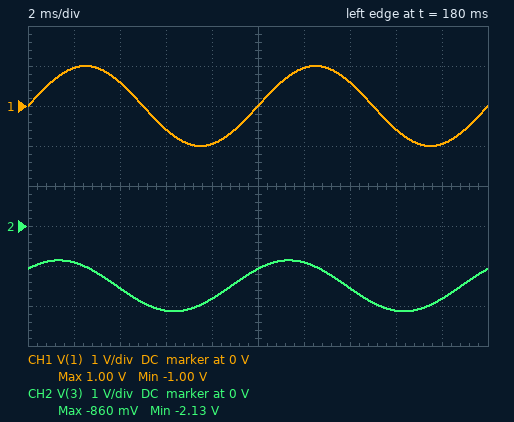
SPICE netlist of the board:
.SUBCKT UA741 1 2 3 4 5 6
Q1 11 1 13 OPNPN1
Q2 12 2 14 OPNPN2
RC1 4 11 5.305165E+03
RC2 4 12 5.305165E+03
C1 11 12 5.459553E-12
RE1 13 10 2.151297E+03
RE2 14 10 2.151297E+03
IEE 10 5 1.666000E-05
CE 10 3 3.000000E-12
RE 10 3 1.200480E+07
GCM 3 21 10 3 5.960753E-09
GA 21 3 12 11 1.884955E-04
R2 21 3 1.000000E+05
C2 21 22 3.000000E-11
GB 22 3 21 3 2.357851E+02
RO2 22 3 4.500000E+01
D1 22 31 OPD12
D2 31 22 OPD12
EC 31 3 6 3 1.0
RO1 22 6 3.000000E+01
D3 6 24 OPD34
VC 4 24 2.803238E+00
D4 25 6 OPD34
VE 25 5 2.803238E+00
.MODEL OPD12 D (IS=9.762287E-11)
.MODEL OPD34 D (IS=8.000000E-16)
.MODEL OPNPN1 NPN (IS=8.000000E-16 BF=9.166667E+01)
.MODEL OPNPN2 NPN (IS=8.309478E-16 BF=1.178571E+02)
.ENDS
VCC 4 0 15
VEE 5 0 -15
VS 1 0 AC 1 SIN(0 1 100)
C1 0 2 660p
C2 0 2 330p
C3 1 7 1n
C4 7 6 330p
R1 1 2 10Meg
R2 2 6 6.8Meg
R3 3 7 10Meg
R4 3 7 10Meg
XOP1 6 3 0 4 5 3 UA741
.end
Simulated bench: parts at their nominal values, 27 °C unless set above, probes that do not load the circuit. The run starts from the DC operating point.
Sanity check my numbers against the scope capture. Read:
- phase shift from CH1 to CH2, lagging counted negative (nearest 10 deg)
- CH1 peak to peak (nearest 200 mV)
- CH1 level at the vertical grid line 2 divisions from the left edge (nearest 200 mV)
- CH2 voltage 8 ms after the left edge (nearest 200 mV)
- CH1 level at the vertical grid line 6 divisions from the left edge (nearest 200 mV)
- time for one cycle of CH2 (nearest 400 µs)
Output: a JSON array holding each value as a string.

["40 deg", "2.0 V", "600 mV", "-1.8 V", "1.0 V", "10.0 ms"]
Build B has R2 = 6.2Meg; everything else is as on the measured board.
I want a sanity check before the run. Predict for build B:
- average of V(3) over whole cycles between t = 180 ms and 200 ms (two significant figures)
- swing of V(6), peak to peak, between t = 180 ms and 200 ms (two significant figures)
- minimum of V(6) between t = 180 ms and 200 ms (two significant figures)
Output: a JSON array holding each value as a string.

["-1.4 V", "1.2 V", "-2.0 V"]
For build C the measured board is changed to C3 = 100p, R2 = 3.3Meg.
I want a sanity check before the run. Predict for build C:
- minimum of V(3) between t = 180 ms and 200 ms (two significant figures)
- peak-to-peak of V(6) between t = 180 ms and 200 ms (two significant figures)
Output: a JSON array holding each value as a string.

["-1.2 V", "26 mV"]
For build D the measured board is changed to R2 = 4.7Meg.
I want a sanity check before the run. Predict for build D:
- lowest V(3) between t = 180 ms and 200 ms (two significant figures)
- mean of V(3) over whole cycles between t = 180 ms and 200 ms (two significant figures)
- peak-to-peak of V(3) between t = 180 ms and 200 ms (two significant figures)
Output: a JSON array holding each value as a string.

["-1.8 V", "-1.3 V", "960 mV"]
